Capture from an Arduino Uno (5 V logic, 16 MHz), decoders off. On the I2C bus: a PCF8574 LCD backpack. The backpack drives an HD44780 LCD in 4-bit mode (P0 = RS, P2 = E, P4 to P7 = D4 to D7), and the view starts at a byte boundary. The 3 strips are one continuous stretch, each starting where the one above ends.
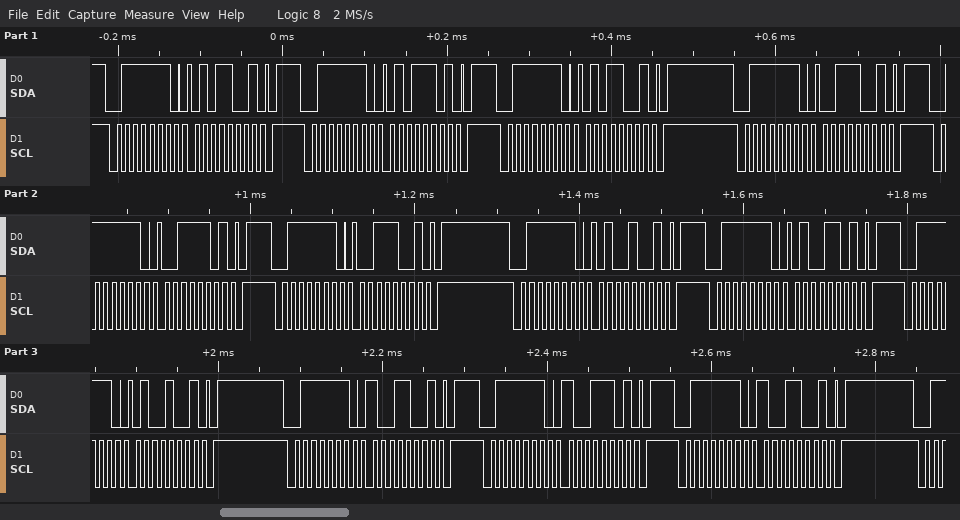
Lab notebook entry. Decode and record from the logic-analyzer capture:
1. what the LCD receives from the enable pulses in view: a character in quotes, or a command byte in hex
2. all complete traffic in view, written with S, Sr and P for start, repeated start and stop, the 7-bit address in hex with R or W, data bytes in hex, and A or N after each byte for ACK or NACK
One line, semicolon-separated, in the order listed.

'S' 'I'; S 3FW A 59 A P S 3FW A 5D A P S 3FW A 59 A P S 3FW A 39 A P S 3FW A 3D A P S 3FW A 39 A P S 3FW A 49 A P S 3FW A 4D A P S 3FW A 49 A P S 3FW A 99 A P S 3FW A 9D A P S 3FW A 99 A P
